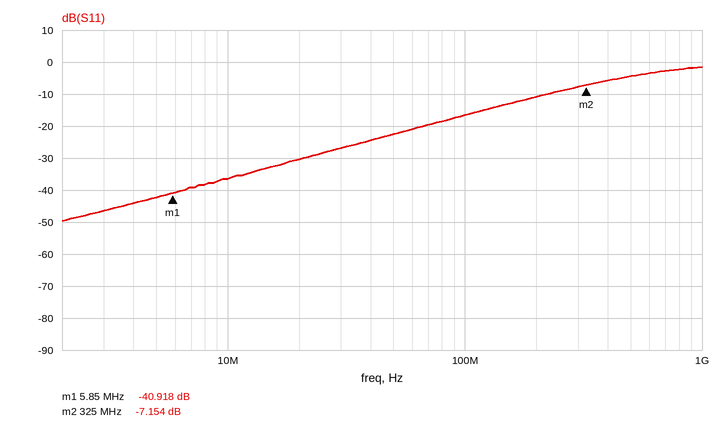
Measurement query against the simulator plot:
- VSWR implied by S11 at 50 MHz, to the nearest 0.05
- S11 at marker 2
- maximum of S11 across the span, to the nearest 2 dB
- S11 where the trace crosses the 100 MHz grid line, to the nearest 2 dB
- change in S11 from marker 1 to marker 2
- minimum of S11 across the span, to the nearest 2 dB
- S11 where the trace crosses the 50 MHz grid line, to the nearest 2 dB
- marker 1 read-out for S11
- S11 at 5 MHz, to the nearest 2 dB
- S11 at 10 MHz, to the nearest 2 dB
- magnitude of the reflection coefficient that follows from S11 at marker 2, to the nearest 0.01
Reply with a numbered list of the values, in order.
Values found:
1. 1.15
2. -7.154 dB
3. -2 dB
4. -16 dB
5. 33.764 dB
6. -50 dB
7. -22 dB
8. -40.918 dB
9. -42 dB
10. -36 dB
11. 0.44
